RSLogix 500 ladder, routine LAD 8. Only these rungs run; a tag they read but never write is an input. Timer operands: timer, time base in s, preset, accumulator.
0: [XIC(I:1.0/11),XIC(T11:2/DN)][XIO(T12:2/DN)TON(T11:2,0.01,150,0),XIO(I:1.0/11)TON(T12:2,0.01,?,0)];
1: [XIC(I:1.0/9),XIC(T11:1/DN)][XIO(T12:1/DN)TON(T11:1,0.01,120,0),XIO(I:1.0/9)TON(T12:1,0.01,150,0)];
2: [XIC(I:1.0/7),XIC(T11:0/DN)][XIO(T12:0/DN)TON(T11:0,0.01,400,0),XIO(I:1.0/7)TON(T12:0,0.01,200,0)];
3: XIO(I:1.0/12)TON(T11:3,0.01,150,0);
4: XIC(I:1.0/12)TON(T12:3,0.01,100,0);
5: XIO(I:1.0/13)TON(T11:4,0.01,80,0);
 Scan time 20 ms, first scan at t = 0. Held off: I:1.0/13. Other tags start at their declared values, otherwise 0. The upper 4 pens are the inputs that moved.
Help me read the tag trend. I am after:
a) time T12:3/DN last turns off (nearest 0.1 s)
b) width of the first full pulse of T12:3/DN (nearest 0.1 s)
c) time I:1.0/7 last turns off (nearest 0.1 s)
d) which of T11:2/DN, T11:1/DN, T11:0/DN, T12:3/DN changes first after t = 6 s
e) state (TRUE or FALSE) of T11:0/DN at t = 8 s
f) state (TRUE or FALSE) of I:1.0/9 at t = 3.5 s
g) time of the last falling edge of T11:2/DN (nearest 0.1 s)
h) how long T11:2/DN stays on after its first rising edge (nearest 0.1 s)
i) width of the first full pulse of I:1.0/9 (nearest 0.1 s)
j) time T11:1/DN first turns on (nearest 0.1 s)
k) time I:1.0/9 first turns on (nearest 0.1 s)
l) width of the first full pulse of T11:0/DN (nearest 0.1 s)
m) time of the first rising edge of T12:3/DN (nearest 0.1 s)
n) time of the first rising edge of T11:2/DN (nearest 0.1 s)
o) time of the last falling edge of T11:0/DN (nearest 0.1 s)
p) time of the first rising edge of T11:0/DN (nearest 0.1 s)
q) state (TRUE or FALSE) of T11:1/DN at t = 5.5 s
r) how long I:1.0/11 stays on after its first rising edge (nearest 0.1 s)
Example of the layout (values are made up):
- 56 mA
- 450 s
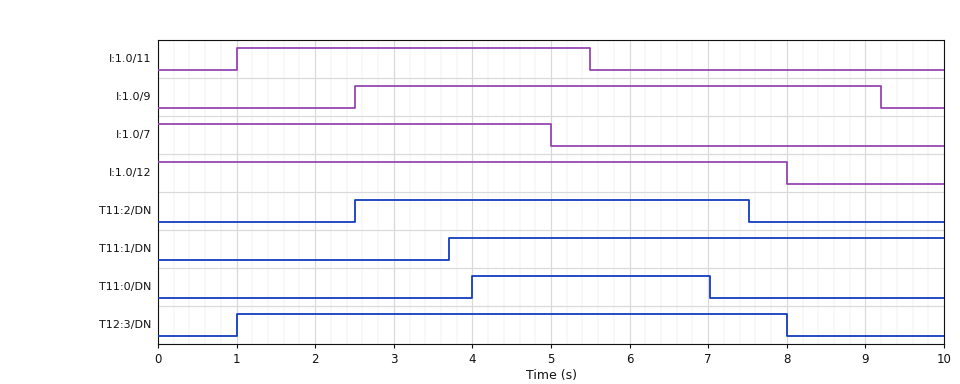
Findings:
- 8.0 s
- 7.0 s
- 5.0 s
- T11:0/DN
- FALSE
- TRUE
- 7.5 s
- 5.0 s
- 6.7 s
- 3.7 s
- 2.5 s
- 3.0 s
- 1.0 s
- 2.5 s
- 7.0 s
- 4.0 s
- TRUE
- 4.5 s
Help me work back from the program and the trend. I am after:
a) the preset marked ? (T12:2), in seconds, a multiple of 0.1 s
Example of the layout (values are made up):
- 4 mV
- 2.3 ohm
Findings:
- 2.0 s
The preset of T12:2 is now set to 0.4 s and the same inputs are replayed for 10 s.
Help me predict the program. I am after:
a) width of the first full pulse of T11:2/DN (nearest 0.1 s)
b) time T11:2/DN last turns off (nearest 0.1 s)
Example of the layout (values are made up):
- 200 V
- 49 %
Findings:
- 3.4 s
- 5.9 s
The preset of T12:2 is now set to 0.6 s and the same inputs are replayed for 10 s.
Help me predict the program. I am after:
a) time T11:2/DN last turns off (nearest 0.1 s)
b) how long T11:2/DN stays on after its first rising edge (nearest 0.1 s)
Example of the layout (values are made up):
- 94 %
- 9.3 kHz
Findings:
- 6.1 s
- 3.6 s
